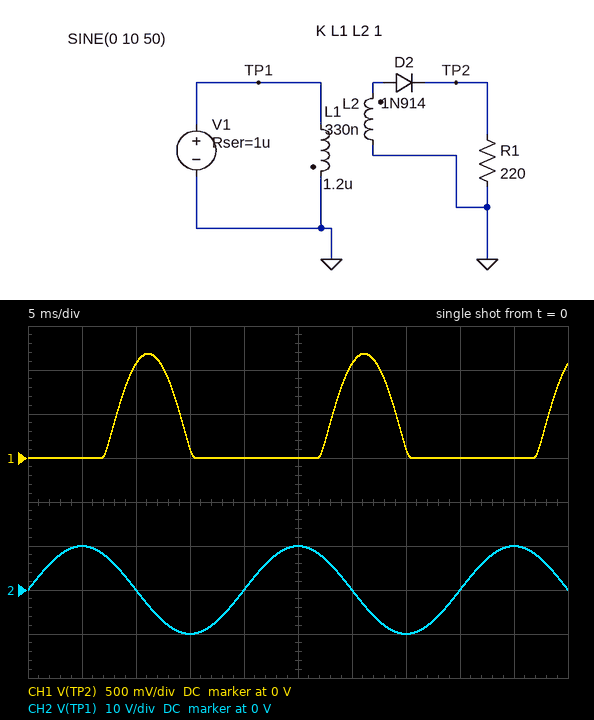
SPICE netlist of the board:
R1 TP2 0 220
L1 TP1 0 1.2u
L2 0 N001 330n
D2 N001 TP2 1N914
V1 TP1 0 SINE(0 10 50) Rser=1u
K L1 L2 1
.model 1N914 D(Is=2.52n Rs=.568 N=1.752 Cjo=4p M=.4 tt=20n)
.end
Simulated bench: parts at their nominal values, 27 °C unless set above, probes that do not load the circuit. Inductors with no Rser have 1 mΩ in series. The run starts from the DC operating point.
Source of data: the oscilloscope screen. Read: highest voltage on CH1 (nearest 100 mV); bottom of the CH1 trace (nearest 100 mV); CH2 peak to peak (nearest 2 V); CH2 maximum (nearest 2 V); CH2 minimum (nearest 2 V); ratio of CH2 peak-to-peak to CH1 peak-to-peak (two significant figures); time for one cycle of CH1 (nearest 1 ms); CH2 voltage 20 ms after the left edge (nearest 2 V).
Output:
1.2 V
0 V
20 V
10 V
-10 V
17
20 ms
0 V
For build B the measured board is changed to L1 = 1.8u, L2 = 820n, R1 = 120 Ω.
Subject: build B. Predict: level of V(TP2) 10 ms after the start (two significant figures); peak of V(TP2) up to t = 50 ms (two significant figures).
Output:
2.2 V
2.6 V
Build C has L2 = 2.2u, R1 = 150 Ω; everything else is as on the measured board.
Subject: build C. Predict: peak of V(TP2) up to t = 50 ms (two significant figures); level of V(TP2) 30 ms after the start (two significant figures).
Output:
4.0 V
3.7 V
